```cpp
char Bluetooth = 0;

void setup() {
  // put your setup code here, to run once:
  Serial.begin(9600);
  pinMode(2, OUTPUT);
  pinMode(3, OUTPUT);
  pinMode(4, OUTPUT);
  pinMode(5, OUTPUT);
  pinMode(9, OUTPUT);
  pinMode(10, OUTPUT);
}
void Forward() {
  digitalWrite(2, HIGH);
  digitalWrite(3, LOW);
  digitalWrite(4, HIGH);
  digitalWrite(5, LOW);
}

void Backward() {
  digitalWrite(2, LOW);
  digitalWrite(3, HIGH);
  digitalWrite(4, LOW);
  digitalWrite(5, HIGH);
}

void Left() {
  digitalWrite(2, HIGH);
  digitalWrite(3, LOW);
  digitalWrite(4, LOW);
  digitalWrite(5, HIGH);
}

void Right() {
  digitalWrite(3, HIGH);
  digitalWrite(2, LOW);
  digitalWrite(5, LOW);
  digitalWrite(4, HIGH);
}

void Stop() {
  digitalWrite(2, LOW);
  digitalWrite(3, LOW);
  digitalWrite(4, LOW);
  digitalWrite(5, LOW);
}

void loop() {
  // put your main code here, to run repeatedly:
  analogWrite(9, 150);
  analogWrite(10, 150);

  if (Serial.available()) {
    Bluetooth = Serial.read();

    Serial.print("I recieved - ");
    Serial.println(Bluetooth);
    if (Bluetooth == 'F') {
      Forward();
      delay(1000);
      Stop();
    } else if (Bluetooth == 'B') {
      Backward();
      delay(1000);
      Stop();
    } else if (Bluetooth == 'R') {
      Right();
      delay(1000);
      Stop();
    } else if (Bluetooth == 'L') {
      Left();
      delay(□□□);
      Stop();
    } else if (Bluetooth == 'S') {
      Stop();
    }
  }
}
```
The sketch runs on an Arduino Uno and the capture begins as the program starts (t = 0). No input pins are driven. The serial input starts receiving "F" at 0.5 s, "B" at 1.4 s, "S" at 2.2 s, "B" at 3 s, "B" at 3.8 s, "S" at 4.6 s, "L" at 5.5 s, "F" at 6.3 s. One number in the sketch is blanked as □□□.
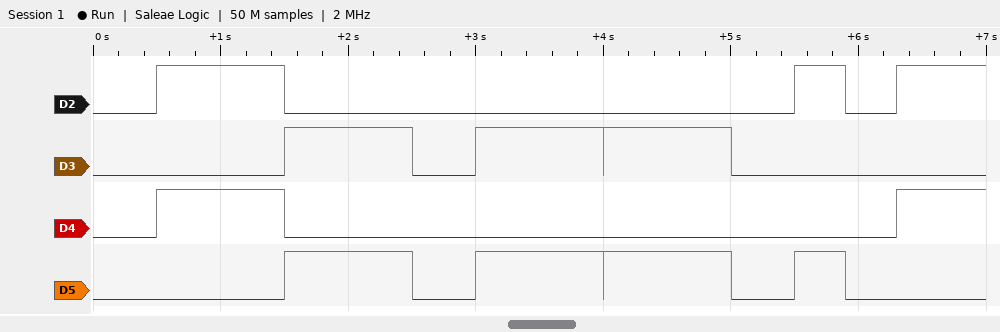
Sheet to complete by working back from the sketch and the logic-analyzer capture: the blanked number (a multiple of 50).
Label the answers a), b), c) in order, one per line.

a) 400
